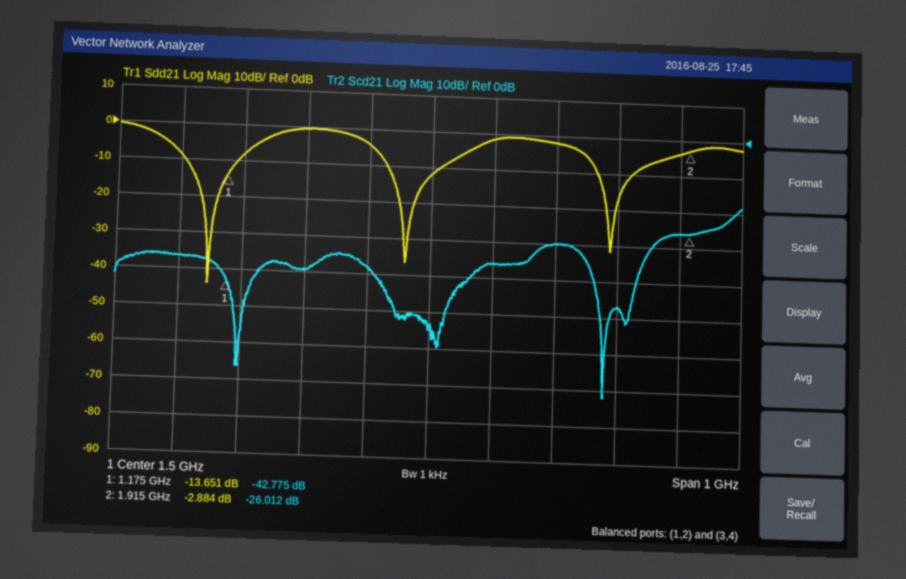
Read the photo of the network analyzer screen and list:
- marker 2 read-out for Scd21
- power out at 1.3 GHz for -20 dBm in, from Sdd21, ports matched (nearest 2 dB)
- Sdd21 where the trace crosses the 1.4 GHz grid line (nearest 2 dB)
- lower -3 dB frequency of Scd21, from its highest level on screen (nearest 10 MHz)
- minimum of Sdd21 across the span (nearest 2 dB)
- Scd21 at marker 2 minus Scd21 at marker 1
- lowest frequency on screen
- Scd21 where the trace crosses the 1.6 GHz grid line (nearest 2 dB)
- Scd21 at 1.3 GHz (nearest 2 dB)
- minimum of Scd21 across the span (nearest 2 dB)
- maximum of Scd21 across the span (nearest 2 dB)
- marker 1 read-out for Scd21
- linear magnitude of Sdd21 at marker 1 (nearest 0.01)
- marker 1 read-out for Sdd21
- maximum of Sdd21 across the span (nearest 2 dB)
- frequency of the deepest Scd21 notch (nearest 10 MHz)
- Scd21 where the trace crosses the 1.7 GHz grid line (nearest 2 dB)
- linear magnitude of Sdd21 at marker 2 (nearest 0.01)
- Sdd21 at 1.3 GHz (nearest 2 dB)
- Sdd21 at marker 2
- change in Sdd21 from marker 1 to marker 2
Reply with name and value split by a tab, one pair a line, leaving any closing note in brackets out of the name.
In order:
marker 2 read-out for Scd21	-26.012 dB
power out at 1.3 GHz for -20 dBm in, from Sdd21, ports matched	-20 dBm
Sdd21 where the trace crosses the 1.4 GHz grid line	-4 dB
lower -3 dB frequency of Scd21, from its highest level on screen	1.98 GHz
minimum of Sdd21 across the span	-44 dB
Scd21 at marker 2 minus Scd21 at marker 1	16.763 dB
lowest frequency on screen	1 GHz
Scd21 where the trace crosses the 1.6 GHz grid line	-36 dB
Scd21 at 1.3 GHz	-40 dB
minimum of Scd21 across the span	-72 dB
maximum of Scd21 across the span	-18 dB
marker 1 read-out for Scd21	-42.775 dB
linear magnitude of Sdd21 at marker 1	0.21
marker 1 read-out for Sdd21	-13.651 dB
maximum of Sdd21 across the span	0 dB
frequency of the deepest Scd21 notch	1.78 GHz
Scd21 where the trace crosses the 1.7 GHz grid line	-30 dB
linear magnitude of Sdd21 at marker 2	0.72
Sdd21 at 1.3 GHz	0 dB
Sdd21 at marker 2	-2.884 dB
change in Sdd21 from marker 1 to marker 2	10.767 dB
